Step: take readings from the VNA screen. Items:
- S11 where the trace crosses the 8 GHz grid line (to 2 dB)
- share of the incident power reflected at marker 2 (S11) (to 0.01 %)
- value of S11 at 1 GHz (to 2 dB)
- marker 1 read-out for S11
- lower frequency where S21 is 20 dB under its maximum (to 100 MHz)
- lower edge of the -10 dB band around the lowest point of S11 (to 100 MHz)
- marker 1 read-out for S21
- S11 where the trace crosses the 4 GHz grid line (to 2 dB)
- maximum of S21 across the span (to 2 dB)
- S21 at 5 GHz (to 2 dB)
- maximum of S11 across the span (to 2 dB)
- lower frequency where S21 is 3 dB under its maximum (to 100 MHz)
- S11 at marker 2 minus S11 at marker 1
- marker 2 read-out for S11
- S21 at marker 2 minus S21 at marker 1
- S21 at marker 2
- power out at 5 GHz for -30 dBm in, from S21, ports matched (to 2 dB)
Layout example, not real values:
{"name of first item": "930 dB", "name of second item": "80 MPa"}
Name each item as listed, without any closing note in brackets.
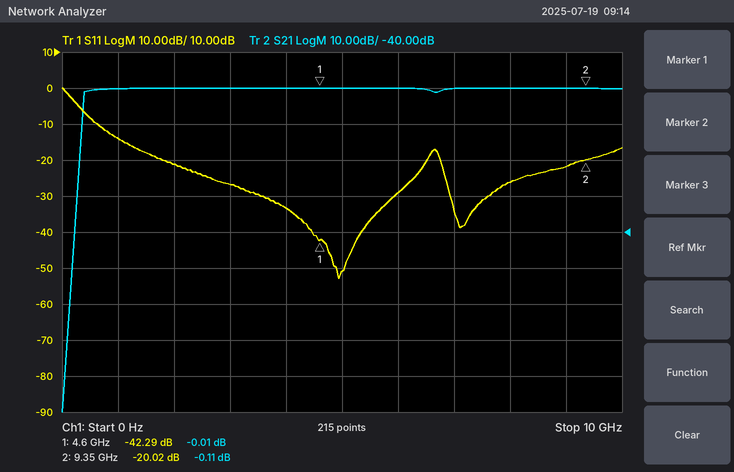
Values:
{"S11 where the trace crosses the 8 GHz grid line": "-26 dB", "share of the incident power reflected at marker 2 (S11)": "1.00 %", "value of S11 at 1 GHz": "-14 dB", "marker 1 read-out for S11": "-42.29 dB", "lower frequency where S21 is 20 dB under its maximum": "300 MHz", "lower edge of the -10 dB band around the lowest point of S11": "600 MHz", "marker 1 read-out for S21": "-0.01 dB", "S11 where the trace crosses the 4 GHz grid line": "-34 dB", "maximum of S21 across the span": "0 dB", "S21 at 5 GHz": "0 dB", "maximum of S11 across the span": "0 dB", "lower frequency where S21 is 3 dB under its maximum": "400 MHz", "S11 at marker 2 minus S11 at marker 1": "22.27 dB", "marker 2 read-out for S11": "-20.02 dB", "S21 at marker 2 minus S21 at marker 1": "-0.10 dB", "S21 at marker 2": "-0.11 dB", "power out at 5 GHz for -30 dBm in, from S21, ports matched": "-30 dBm"}
